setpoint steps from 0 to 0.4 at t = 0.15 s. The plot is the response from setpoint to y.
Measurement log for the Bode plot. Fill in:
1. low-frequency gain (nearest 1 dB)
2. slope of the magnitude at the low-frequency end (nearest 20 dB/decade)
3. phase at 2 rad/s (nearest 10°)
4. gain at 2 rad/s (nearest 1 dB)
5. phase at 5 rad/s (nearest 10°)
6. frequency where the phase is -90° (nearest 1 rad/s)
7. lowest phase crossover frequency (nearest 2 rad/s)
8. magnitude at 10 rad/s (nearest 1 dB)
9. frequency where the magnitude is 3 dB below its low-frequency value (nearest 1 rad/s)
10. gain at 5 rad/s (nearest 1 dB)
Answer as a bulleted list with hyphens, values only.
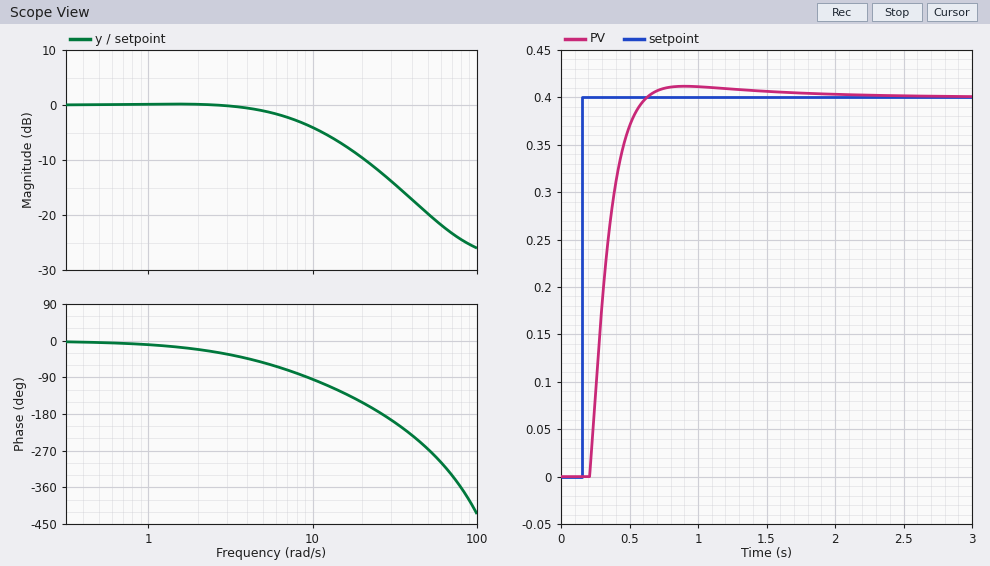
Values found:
- 0 dB
- 0 dB/decade
- -20°
- 0 dB
- -50°
- 9 rad/s
- 26 rad/s
- -4 dB
- 8 rad/s
- -1 dB
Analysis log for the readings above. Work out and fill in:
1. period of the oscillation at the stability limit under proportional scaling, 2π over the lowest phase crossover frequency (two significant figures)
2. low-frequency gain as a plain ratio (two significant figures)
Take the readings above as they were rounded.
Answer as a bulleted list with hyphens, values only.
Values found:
- 0.24 s
- 1.0
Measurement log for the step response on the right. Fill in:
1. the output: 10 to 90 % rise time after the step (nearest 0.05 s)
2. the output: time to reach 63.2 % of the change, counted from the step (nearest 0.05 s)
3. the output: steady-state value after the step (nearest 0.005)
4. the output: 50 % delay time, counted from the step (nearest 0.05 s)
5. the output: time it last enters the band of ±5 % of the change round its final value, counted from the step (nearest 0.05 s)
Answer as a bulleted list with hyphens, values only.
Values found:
- 0.25 s
- 0.20 s
- 0.400
- 0.15 s
- 0.40 s
